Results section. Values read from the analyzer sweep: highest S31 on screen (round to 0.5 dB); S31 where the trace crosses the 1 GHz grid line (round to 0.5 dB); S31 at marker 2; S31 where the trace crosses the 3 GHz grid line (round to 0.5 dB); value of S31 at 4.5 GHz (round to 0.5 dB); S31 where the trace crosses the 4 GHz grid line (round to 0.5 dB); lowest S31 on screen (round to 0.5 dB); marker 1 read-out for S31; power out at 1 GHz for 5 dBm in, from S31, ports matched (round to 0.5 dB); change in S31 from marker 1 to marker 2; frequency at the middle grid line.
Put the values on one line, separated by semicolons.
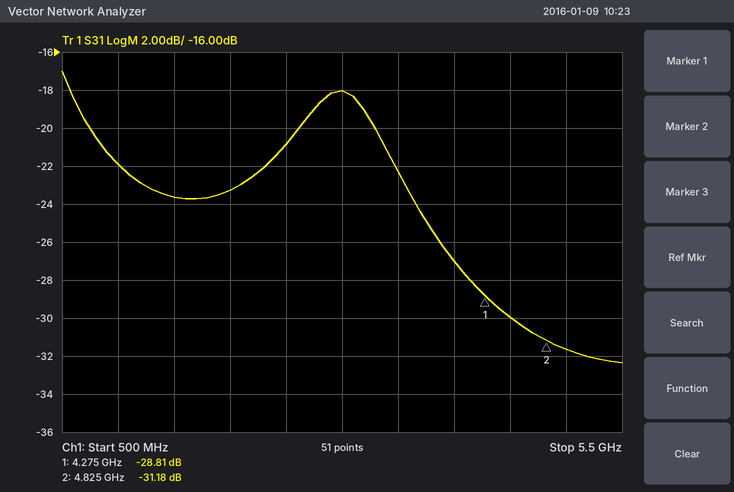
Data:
-17.0 dB; -22.0 dB; -31.18 dB; -18.0 dB; -30.0 dB; -27.0 dB; -32.5 dB; -28.81 dB; -17.0 dBm; -2.37 dB; 3 GHz
